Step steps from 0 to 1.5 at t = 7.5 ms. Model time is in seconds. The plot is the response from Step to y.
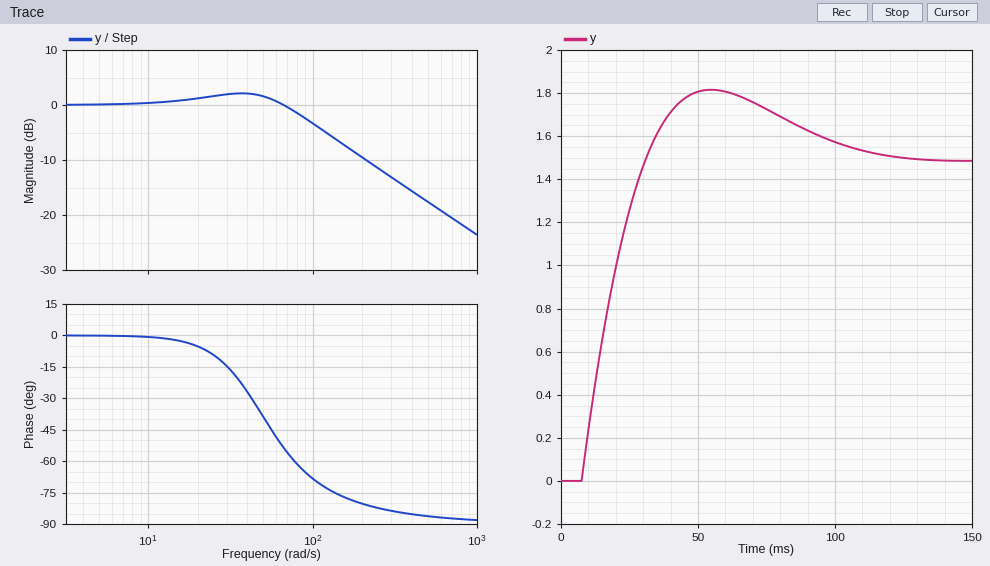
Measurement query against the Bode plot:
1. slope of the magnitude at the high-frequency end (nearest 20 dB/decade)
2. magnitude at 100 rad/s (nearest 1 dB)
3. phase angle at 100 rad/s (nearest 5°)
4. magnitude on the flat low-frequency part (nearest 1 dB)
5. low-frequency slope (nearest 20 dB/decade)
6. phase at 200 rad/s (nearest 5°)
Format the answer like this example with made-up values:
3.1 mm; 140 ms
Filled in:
-20 dB/decade; -3 dB; -70°; 0 dB; 0 dB/decade; -80°
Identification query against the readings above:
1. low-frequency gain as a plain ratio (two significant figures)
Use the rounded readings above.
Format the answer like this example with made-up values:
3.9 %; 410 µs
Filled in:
1.0
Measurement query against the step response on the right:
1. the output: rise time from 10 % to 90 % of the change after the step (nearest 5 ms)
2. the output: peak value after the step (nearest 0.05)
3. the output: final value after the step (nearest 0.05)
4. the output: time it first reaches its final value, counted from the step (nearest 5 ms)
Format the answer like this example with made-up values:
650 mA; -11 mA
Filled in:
20 ms; 1.80; 1.50; 25 ms
